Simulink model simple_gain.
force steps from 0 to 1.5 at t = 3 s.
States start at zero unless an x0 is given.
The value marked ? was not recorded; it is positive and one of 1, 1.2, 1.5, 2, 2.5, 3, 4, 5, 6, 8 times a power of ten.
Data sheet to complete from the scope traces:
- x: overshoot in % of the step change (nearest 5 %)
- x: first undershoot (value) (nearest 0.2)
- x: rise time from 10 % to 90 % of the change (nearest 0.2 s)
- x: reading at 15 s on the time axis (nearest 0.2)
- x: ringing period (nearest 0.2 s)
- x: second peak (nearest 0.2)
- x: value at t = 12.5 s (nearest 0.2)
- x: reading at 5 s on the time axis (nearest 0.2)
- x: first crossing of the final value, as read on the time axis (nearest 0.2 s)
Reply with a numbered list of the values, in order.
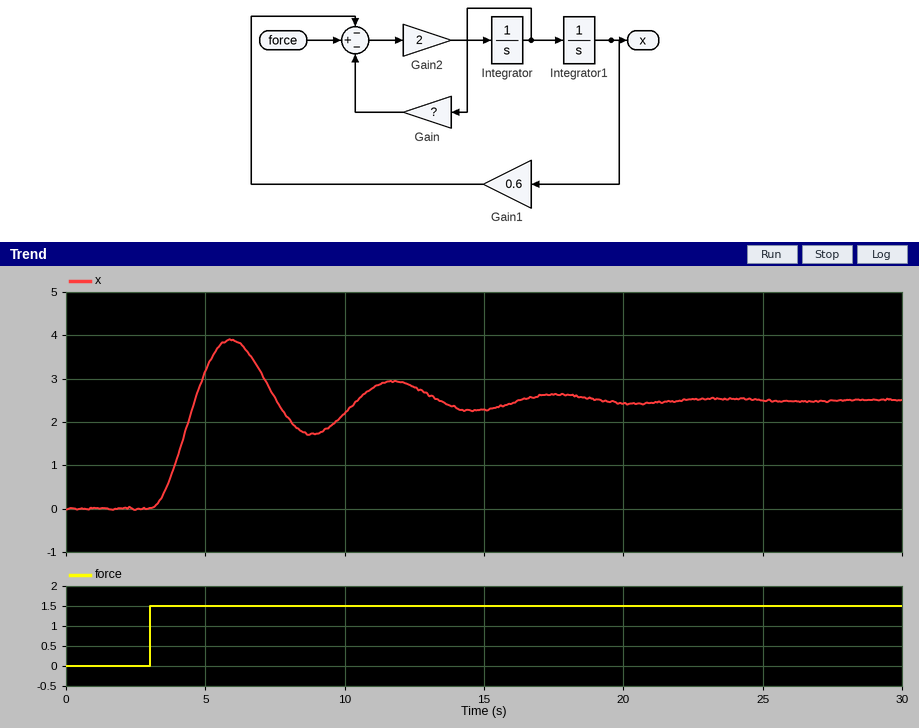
1. 55 %
2. 1.8
3. 1.0 s
4. 2.2
5. 5.8 s
6. 3.0
7. 2.8
8. 3.2
9. 4.6 s
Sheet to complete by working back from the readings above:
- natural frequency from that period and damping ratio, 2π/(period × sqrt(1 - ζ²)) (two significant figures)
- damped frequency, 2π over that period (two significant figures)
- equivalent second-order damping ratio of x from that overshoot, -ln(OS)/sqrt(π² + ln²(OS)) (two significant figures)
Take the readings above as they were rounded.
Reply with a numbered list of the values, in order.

1. 1.1 rad/s
2. 1.1 rad/s
3. 0.19
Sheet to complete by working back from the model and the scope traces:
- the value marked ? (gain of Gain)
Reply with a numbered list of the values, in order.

1. 0.2
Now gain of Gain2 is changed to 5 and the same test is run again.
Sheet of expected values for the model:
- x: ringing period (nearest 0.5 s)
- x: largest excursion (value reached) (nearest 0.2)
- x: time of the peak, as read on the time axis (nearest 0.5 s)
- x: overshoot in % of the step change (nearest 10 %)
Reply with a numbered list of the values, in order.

1. 4.0 s
2. 3.4
3. 5.0 s
4. 40 %
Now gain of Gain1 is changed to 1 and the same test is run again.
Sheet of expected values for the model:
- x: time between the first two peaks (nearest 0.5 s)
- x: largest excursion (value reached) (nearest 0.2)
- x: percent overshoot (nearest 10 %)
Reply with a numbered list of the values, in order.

1. 4.5 s
2. 2.4
3. 60 %
